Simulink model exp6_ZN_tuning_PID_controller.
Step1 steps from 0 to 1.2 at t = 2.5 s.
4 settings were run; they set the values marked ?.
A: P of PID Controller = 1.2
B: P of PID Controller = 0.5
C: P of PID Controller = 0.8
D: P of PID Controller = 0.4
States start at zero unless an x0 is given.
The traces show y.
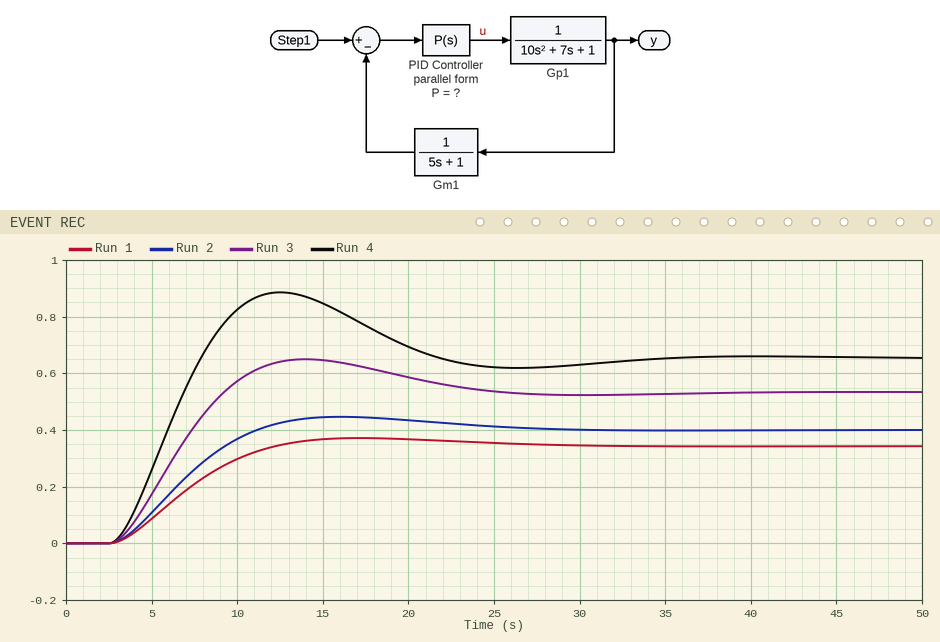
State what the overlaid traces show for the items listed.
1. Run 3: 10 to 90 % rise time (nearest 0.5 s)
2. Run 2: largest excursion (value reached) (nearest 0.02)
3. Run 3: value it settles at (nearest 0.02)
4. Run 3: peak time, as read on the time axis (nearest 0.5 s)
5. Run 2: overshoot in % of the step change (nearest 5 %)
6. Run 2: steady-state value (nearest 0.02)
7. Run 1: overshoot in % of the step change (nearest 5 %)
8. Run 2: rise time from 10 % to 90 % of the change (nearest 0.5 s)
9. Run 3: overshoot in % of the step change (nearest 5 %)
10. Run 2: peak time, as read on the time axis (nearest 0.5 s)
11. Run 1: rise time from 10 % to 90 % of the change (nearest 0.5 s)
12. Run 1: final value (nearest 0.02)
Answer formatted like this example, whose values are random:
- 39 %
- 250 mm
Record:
- 4.5 s
- 0.44
- 0.54
- 14.0 s
- 10 %
- 0.40
- 10 %
- 6.0 s
- 20 %
- 16.0 s
- 6.5 s
- 0.34
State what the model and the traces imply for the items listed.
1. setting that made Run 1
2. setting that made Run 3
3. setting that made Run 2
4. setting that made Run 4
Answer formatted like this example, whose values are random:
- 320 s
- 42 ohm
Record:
- D
- C
- B
- A
